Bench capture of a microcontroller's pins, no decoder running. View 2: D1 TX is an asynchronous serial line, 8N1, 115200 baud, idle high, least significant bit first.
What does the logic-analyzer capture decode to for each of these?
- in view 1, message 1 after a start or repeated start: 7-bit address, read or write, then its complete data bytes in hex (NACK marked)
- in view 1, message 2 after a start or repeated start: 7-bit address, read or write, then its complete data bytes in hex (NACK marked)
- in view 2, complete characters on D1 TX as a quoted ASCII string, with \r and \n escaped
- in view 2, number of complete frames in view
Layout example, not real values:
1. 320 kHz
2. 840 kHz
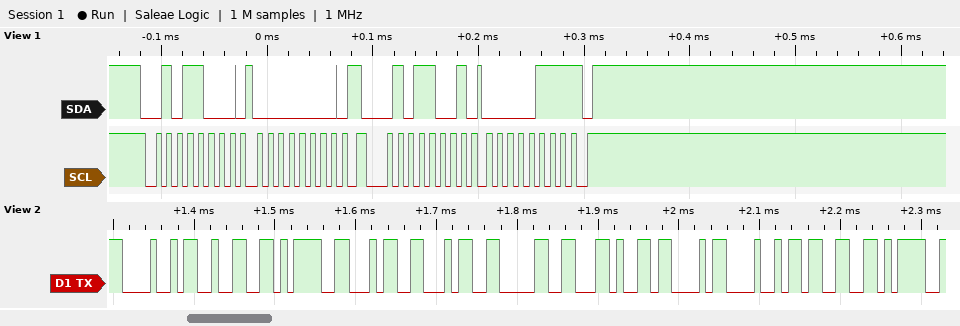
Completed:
1. 0x2C write: 00
2. 0x2C read: 07 NACK
3. "H2=440,CH3="
4. 11
